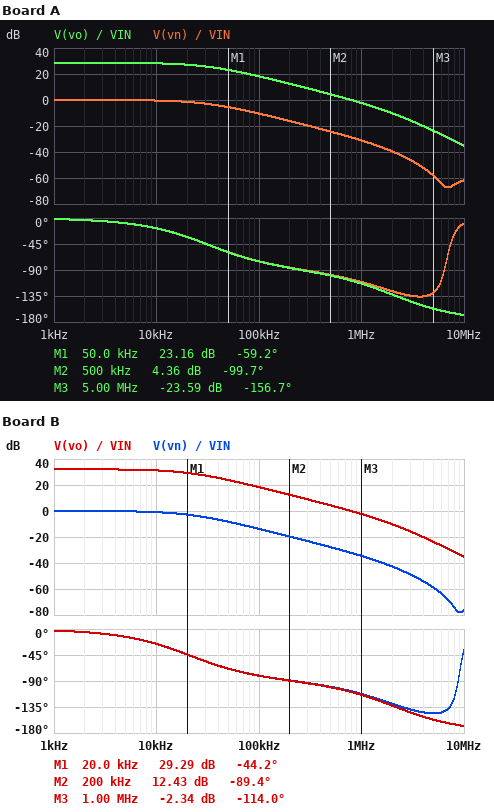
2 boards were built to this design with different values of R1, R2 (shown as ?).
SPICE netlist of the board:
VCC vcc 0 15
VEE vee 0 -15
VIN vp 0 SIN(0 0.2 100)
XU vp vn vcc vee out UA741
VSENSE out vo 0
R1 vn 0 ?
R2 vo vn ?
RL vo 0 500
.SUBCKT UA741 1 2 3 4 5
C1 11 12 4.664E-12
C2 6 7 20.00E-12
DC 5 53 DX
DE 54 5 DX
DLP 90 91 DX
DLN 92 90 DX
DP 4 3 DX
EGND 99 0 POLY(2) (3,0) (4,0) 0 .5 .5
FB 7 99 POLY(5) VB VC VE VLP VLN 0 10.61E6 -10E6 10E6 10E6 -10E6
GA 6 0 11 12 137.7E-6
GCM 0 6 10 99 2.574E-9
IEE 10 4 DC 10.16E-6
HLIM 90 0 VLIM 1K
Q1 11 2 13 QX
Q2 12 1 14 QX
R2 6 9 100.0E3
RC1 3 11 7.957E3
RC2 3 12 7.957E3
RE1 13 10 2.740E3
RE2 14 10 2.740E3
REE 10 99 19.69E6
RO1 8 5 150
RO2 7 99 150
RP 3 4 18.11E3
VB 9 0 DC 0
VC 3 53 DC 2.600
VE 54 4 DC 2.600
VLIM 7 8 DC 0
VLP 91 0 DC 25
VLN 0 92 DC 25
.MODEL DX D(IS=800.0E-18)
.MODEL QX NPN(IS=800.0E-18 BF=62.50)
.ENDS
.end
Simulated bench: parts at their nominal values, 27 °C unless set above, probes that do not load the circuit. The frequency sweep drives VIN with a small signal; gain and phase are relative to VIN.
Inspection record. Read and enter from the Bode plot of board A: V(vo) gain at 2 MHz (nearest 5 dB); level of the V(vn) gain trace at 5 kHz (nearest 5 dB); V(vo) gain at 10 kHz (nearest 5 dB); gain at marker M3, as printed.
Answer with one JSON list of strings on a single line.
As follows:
["-10 dB", "0 dB", "30 dB", "-23.59 dB"]
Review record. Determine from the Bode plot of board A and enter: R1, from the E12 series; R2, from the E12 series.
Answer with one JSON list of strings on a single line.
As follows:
["1.5 kΩ", "39 kΩ"]
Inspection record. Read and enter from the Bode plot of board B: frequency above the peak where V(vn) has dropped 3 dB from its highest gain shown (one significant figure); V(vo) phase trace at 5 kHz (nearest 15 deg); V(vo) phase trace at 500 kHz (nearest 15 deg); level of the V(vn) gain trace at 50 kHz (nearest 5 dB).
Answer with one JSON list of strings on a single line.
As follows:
["20 kHz", "-15 deg", "-105 deg", "-10 dB"]
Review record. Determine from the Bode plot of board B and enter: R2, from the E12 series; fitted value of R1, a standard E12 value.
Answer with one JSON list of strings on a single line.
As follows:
["22 kΩ", "560 Ω"]
